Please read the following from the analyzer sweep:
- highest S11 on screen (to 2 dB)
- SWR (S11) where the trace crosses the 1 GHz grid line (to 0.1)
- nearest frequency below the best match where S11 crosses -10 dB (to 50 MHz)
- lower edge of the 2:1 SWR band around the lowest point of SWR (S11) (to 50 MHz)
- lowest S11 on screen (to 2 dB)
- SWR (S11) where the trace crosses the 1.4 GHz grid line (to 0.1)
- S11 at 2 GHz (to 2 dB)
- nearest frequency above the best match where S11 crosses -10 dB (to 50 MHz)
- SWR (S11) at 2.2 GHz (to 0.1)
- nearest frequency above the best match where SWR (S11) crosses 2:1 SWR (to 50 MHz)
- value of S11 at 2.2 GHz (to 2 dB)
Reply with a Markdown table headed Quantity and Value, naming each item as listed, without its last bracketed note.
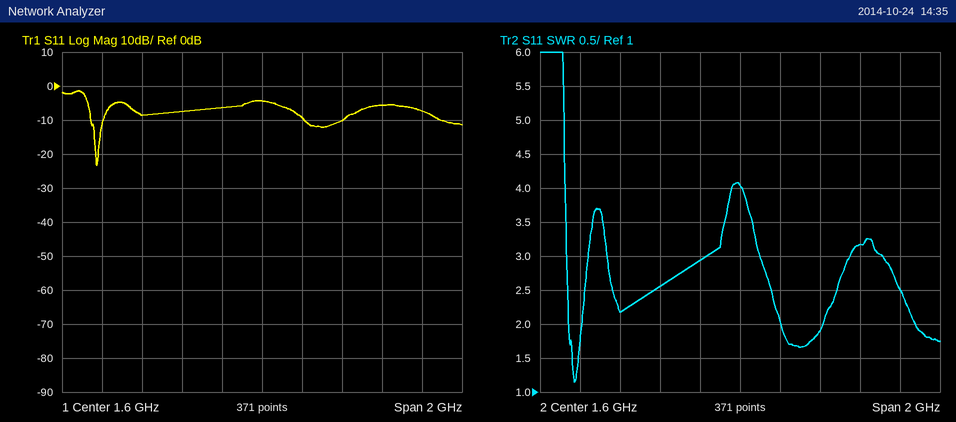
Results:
| Quantity | Value |
|---|---|
| highest S11 on screen | -2 dB |
| SWR (S11) where the trace crosses the 1 GHz grid line | 2.2 |
| nearest frequency below the best match where S11 crosses -10 dB | 750 MHz |
| lower edge of the 2:1 SWR band around the lowest point of SWR (S11) | 750 MHz |
| lowest S11 on screen | -24 dB |
| SWR (S11) where the trace crosses the 1.4 GHz grid line | 2.9 |
| S11 at 2 GHz | -10 dB |
| nearest frequency above the best match where S11 crosses -10 dB | 800 MHz |
| SWR (S11) at 2.2 GHz | 3.2 |
| nearest frequency above the best match where SWR (S11) crosses 2:1 SWR | 800 MHz |
| value of S11 at 2.2 GHz | -6 dB |
